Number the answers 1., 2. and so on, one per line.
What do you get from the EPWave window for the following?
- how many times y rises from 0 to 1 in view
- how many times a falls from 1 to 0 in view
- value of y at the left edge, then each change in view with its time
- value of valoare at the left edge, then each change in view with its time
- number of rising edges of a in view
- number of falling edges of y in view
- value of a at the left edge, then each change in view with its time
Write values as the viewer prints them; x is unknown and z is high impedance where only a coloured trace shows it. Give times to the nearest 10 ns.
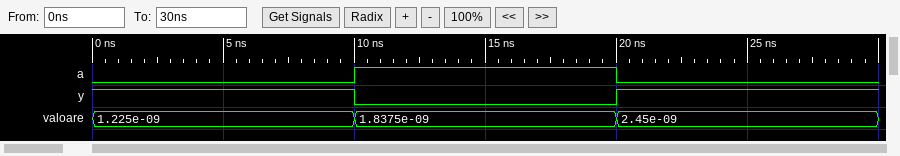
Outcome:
1. 1
2. 1
3. 1, 0 at 10 ns, 1 at 20 ns
4. 1.225e-09, 1.8375e-09 at 10 ns, 2.45e-09 at 20 ns
5. 1
6. 1
7. 0, 1 at 10 ns, 0 at 20 ns
